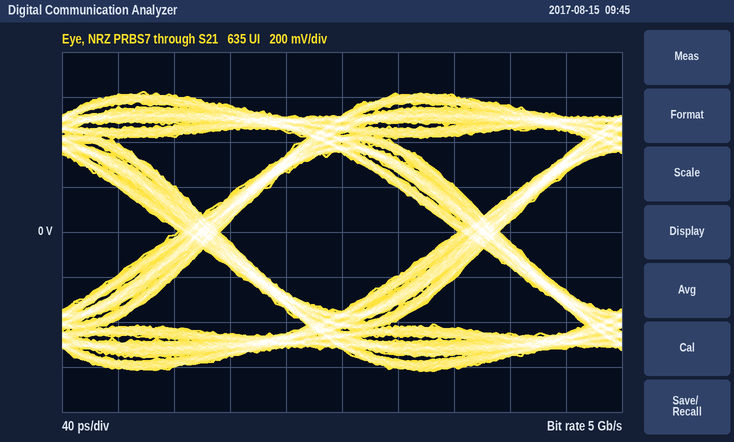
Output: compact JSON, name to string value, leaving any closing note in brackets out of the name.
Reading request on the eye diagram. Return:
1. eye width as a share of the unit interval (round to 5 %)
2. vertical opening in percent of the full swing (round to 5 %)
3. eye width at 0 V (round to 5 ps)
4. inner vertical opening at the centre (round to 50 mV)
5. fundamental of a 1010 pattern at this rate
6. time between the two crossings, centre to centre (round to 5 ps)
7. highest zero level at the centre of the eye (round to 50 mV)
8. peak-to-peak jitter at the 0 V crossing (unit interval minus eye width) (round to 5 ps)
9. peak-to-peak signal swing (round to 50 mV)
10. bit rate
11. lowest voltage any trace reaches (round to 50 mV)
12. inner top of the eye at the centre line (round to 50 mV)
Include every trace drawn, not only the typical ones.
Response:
{"eye width as a share of the unit interval": "85 %", "vertical opening in percent of the full swing": "55 %", "eye width at 0 V": "170 ps", "inner vertical opening at the centre": "700 mV", "fundamental of a 1010 pattern at this rate": "2.5 GHz", "time between the two crossings, centre to centre": "200 ps", "highest zero level at the centre of the eye": "-350 mV", "peak-to-peak jitter at the 0 V crossing (unit interval minus eye width)": "30 ps", "peak-to-peak signal swing": "1.25 V", "bit rate": "5 Gb/s", "lowest voltage any trace reaches": "-600 mV", "inner top of the eye at the centre line": "350 mV"}
